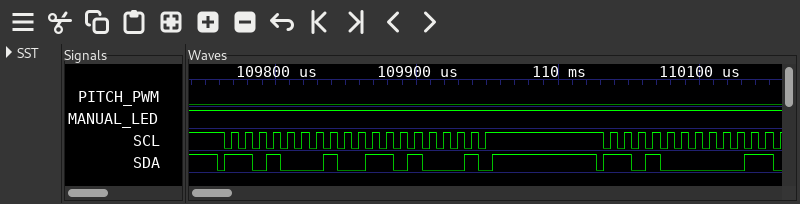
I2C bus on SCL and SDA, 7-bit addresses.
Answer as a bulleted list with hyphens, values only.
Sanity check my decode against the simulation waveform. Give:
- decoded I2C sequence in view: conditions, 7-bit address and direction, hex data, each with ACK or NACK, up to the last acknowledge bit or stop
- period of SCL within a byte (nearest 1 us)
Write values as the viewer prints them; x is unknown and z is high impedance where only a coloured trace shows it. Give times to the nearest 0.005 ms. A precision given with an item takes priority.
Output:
- start, address 68 read ACK, 68 NACK, stop, start, address 68 write ACK
- 10 us
